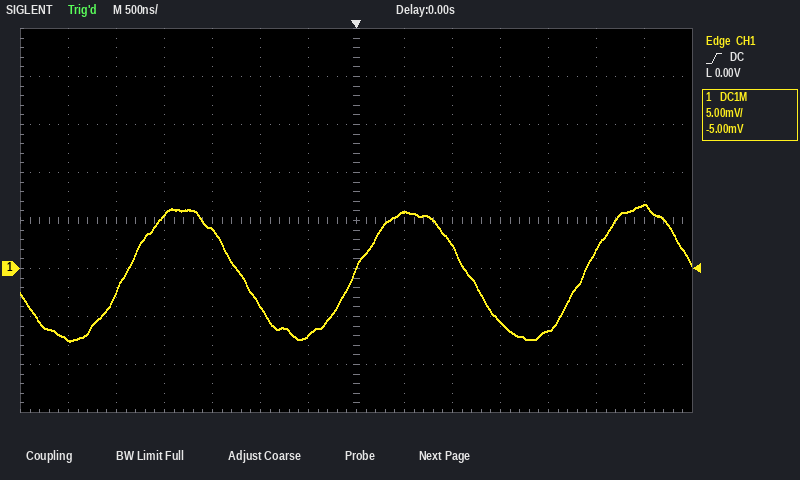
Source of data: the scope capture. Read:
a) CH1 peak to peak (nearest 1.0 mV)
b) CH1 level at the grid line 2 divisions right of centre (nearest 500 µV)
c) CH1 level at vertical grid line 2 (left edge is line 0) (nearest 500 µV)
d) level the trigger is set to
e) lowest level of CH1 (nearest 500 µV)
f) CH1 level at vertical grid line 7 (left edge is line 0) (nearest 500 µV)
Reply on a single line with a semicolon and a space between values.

14.0 mV; 2.5 mV; -2.5 mV; 0.00 V; -7.5 mV; 0.0 mV
